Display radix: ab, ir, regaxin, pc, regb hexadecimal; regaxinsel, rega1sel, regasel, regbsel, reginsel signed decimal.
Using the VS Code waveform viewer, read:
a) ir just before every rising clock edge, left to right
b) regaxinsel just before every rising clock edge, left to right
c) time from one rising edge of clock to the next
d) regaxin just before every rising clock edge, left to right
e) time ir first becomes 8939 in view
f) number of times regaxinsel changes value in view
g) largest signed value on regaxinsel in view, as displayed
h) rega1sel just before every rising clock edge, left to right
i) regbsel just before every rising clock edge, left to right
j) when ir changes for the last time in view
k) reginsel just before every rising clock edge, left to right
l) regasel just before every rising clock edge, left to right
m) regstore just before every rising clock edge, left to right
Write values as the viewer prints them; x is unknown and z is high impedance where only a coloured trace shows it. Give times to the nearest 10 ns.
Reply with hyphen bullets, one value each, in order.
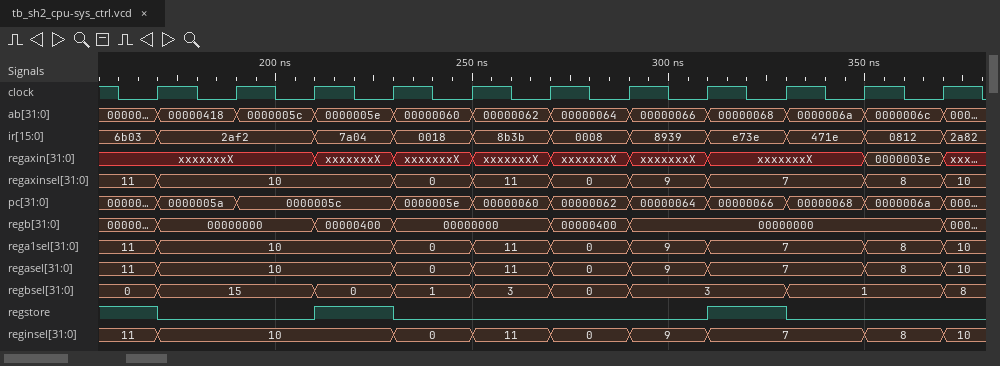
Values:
- 6b03, 2af2, 2af2, 7a04, 0018, 8b3b, 0008, 8939, e73e, 471e, 0812
- 11, 10, 10, 10, 0, 11, 0, 9, 7, 7, 8
- 20 ns
- xxxxxxxX, xxxxxxxX, xxxxxxxX, xxxxxxxX, xxxxxxxX, xxxxxxxX, xxxxxxxX, xxxxxxxX, xxxxxxxX, xxxxxxxX, 0000003e
- 290 ns
- 8
- 11
- 11, 10, 10, 10, 0, 11, 0, 9, 7, 7, 8
- 0, 15, 15, 0, 1, 3, 0, 3, 3, 1, 1
- 370 ns
- 11, 10, 10, 10, 0, 11, 0, 9, 7, 7, 8
- 11, 10, 10, 10, 0, 11, 0, 9, 7, 7, 8
- 1 0 0 1 0 0 0 0 1 0 0
